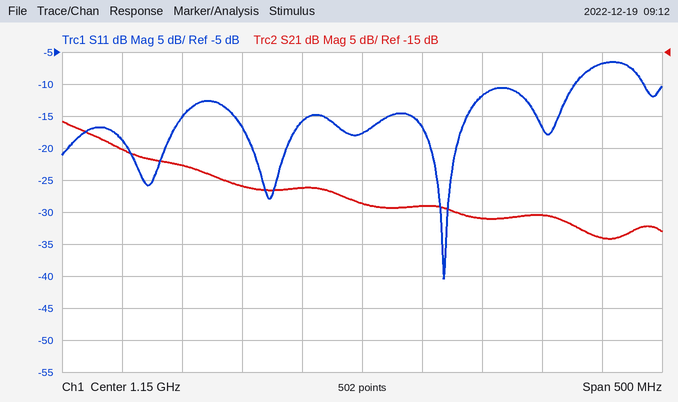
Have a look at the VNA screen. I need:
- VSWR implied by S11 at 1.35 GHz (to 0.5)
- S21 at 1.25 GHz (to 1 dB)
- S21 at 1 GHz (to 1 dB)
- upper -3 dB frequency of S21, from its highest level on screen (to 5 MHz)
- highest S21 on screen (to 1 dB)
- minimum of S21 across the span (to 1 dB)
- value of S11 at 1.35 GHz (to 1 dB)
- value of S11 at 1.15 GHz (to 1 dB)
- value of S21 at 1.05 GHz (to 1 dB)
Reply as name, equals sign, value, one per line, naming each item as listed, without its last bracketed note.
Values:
VSWR implied by S11 at 1.35 GHz = 2.5
S21 at 1.25 GHz = -41 dB
S21 at 1 GHz = -33 dB
upper -3 dB frequency of S21, from its highest level on screen = 935 MHz
highest S21 on screen = -26 dB
minimum of S21 across the span = -44 dB
value of S11 at 1.35 GHz = -7 dB
value of S11 at 1.15 GHz = -18 dB
value of S21 at 1.05 GHz = -36 dB
